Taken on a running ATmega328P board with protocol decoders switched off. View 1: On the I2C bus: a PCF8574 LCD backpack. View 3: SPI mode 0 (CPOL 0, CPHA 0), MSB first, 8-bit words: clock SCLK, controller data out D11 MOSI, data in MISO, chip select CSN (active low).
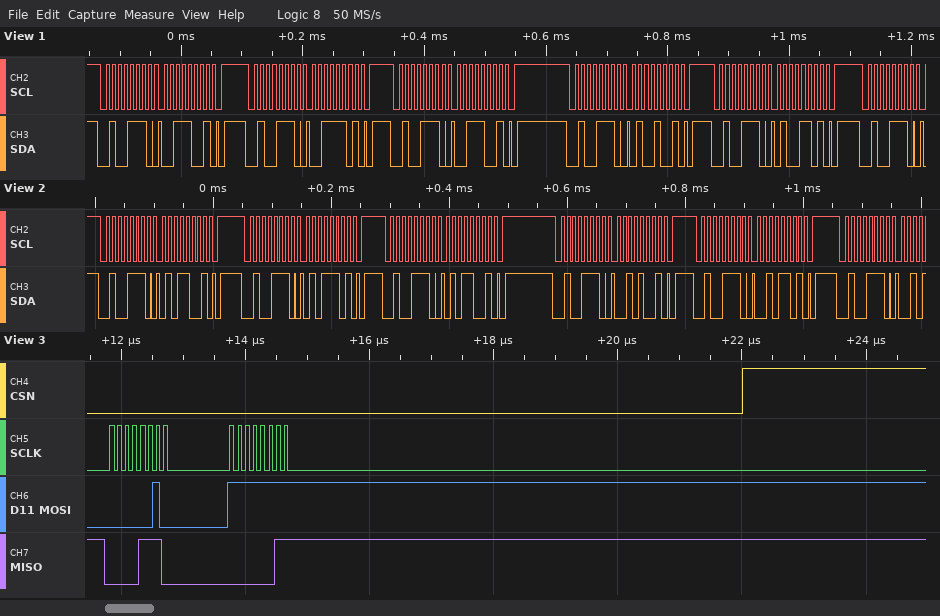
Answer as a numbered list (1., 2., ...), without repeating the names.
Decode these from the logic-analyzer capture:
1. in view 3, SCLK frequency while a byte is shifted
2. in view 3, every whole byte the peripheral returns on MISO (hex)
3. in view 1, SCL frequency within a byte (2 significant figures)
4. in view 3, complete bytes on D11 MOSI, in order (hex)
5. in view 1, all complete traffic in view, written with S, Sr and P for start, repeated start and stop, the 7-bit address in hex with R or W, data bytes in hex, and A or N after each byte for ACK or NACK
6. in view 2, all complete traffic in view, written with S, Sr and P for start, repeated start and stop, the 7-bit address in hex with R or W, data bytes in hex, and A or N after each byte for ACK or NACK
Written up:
1. 8 MHz
2. 0E 03
3. 100 kHz
4. 02 FF
5. S 27W A 39 A P S 27W A 3D A P S 27W A 39 A P S 27W A 49 A P S 27W A 4D A P S 27W A
6. S 27W A 59 A P S 27W A 5D A P S 27W A 59 A P S 27W A 29 A P S 27W A 2D A P S 27W A
